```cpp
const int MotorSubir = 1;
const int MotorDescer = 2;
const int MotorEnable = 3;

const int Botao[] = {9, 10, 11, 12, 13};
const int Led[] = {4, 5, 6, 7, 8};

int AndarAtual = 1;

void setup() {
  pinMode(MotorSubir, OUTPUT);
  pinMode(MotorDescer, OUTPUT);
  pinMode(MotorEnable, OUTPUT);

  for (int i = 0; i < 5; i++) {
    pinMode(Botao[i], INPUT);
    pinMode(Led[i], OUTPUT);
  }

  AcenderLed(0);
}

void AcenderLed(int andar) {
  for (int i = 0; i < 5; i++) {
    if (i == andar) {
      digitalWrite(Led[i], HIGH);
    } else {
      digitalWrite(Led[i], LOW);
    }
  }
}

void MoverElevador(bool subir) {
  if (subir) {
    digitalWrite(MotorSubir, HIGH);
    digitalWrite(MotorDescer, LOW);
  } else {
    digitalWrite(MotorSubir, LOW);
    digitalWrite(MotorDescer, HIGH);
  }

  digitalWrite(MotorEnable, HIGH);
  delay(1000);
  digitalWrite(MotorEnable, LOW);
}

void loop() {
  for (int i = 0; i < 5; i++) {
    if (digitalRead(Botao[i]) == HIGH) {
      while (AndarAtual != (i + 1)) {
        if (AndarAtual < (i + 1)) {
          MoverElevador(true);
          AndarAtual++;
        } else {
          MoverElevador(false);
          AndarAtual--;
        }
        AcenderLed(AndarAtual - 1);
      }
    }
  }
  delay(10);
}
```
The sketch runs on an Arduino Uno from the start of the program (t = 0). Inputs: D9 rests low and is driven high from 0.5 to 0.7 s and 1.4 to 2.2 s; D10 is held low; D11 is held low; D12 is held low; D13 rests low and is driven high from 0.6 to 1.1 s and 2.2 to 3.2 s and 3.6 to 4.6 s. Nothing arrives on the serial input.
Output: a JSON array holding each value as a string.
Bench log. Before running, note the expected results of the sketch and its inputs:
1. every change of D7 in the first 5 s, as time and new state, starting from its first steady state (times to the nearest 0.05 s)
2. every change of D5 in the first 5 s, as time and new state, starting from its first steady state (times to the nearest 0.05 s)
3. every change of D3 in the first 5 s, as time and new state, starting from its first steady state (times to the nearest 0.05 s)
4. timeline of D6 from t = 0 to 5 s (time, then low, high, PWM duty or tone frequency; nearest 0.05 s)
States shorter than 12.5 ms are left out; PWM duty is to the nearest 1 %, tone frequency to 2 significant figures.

["0 s low; 3.6 s high; 4.6 s low", "0 s low; 1.6 s high; 2.6 s low", "0 s low; 0.6 s high; 4.6 s low", "0 s low; 2.6 s high; 3.6 s low"]
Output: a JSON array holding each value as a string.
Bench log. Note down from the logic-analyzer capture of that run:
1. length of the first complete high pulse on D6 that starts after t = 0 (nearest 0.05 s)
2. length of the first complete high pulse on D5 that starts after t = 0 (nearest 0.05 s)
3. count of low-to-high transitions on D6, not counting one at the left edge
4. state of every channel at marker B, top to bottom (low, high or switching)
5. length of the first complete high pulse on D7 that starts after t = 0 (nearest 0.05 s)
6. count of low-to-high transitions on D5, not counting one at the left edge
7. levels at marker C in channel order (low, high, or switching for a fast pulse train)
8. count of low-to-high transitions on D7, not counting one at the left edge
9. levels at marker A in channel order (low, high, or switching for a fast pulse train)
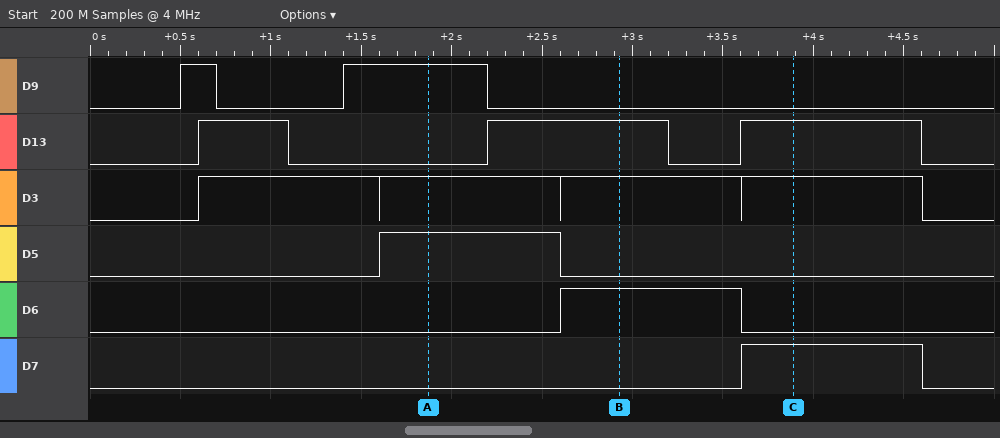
["1.00 s", "1.00 s", "1", "D9 low, D13 high, D3 high, D5 low, D6 high, D7 low", "1.00 s", "1", "D9 low, D13 high, D3 high, D5 low, D6 low, D7 high", "1", "D9 high, D13 low, D3 high, D5 high, D6 low, D7 low"]
